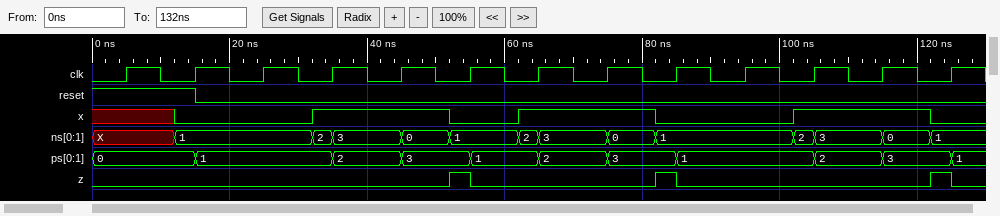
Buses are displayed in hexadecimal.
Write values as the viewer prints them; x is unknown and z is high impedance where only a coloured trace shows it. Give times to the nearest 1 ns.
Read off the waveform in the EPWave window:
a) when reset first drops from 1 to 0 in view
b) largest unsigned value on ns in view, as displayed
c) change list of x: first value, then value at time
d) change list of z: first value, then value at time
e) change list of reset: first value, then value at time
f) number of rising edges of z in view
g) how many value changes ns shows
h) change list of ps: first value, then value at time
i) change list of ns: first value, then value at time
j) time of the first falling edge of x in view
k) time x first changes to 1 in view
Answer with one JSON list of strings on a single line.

["15 ns", "3", "x, 0 at 12 ns, 1 at 32 ns, 0 at 52 ns, 1 at 62 ns, 0 at 82 ns, 1 at 102 ns, 0 at 122 ns", "0, 1 at 52 ns, 0 at 55 ns, 1 at 82 ns, 0 at 85 ns, 1 at 122 ns, 0 at 125 ns", "1, 0 at 15 ns", "3", "13", "0, 1 at 15 ns, 2 at 35 ns, 3 at 45 ns, 1 at 55 ns, 2 at 65 ns, 3 at 75 ns, 1 at 85 ns, 2 at 105 ns, 3 at 115 ns, 1 at 125 ns", "X, 1 at 12 ns, 2 at 32 ns, 3 at 35 ns, 0 at 45 ns, 1 at 52 ns, 2 at 62 ns, 3 at 65 ns, 0 at 75 ns, 1 at 82 ns, 2 at 102 ns, 3 at 105 ns, 0 at 115 ns, 1 at 122 ns", "52 ns", "32 ns"]
